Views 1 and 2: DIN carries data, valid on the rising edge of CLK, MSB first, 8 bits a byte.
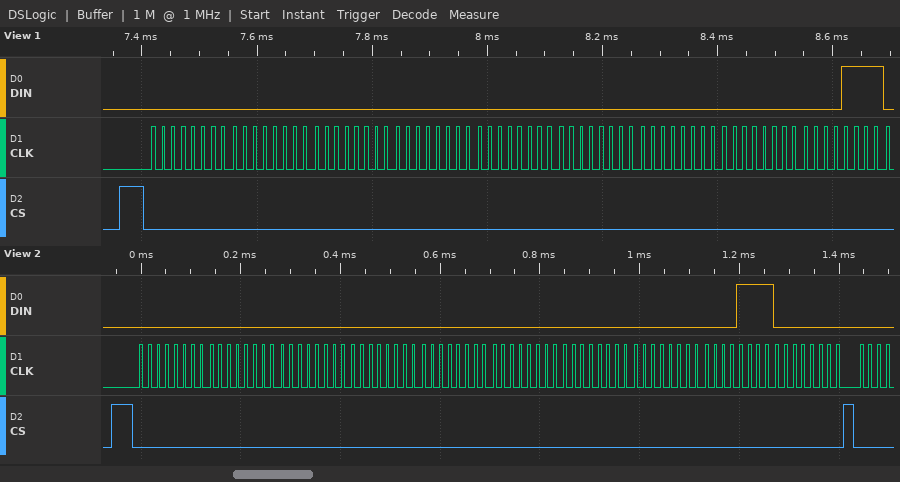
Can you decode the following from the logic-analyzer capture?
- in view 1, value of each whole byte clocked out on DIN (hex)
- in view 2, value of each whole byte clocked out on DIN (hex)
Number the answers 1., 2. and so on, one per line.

1. 00 00 00 00 00 00 00 00 0F
2. 00 00 00 00 00 00 00 00 0F 00
